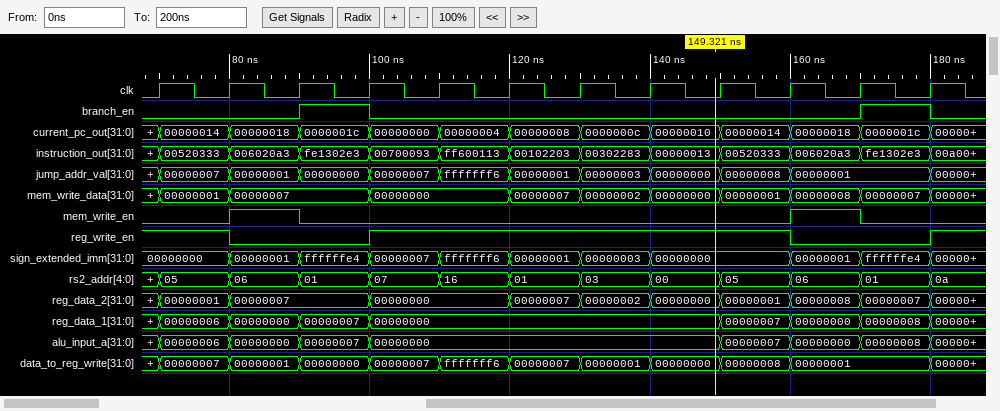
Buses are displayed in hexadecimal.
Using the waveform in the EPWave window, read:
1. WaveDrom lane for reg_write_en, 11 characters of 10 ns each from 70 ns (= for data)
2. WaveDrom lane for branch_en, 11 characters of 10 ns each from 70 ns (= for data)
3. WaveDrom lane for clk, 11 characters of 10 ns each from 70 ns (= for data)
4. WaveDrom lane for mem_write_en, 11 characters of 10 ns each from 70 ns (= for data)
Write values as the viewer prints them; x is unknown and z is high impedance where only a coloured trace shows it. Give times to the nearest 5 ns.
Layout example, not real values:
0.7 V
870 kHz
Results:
{name: 'reg_write_en', wave: '10.1.....0.'}
{name: 'branch_en', wave: '0.10......1'}
{name: 'clk', wave: 'p..........'}
{name: 'mem_write_en', wave: '010......10'}
